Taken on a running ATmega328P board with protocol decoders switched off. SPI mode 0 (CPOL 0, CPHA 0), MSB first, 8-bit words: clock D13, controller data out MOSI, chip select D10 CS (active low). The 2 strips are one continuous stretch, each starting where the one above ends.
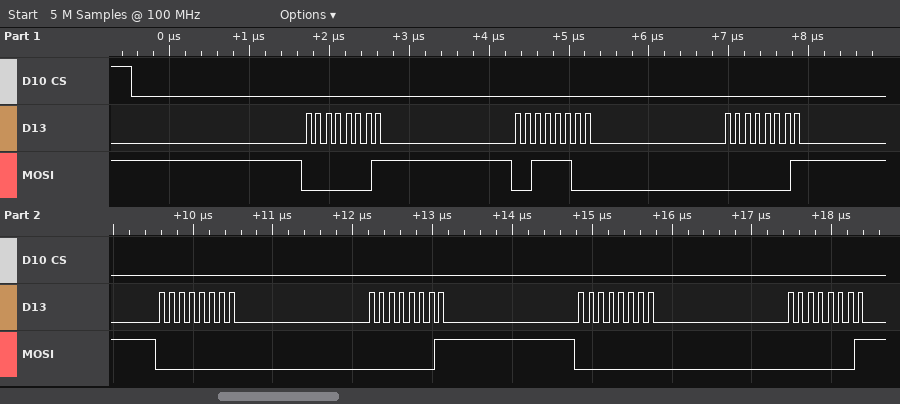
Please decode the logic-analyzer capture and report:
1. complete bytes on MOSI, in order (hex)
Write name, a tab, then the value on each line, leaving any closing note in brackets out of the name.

complete bytes on MOSI, in order	01 3C 01 00 01 00 01
